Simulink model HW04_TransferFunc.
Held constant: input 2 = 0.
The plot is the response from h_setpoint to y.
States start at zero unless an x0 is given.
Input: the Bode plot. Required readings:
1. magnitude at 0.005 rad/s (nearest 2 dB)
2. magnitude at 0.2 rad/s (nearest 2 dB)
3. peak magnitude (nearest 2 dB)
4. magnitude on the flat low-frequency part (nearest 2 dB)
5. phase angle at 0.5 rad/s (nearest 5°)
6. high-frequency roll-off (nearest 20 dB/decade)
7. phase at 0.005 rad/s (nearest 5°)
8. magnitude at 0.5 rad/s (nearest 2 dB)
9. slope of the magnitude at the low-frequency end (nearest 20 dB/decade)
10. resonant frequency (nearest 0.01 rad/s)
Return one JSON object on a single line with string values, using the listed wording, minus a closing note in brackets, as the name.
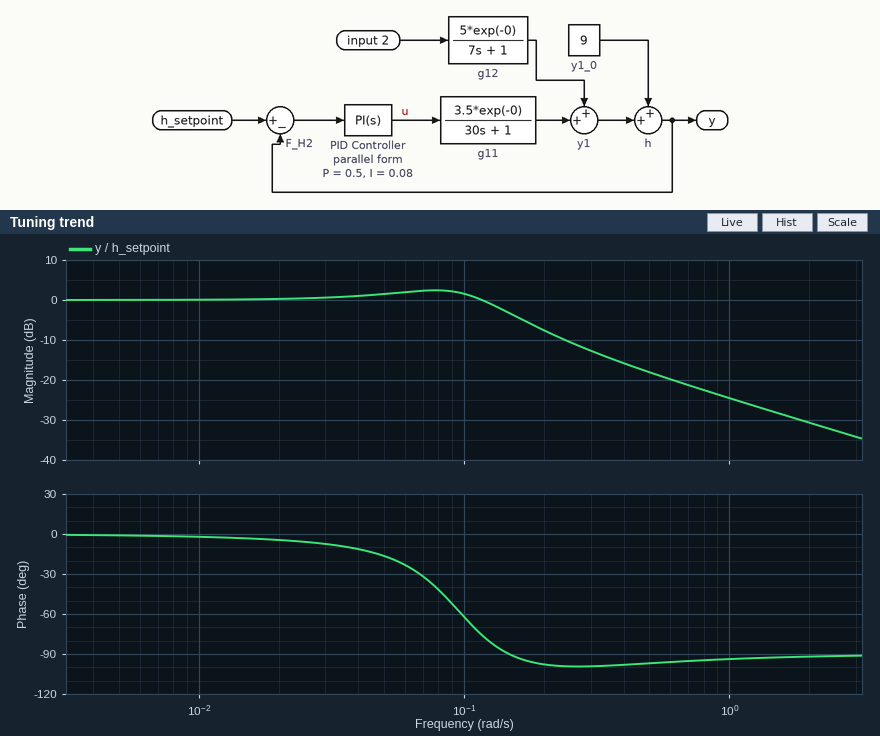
{"magnitude at 0.005 rad/s": "0 dB", "magnitude at 0.2 rad/s": "-8 dB", "peak magnitude": "2 dB", "magnitude on the flat low-frequency part": "0 dB", "phase angle at 0.5 rad/s": "-95°", "high-frequency roll-off": "-20 dB/decade", "phase at 0.005 rad/s": "0°", "magnitude at 0.5 rad/s": "-18 dB", "slope of the magnitude at the low-frequency end": "0 dB/decade", "resonant frequency": "0.08 rad/s"}
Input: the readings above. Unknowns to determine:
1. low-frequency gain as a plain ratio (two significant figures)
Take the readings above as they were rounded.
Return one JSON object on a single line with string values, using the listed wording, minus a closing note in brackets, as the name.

{"low-frequency gain as a plain ratio": "1.0"}
